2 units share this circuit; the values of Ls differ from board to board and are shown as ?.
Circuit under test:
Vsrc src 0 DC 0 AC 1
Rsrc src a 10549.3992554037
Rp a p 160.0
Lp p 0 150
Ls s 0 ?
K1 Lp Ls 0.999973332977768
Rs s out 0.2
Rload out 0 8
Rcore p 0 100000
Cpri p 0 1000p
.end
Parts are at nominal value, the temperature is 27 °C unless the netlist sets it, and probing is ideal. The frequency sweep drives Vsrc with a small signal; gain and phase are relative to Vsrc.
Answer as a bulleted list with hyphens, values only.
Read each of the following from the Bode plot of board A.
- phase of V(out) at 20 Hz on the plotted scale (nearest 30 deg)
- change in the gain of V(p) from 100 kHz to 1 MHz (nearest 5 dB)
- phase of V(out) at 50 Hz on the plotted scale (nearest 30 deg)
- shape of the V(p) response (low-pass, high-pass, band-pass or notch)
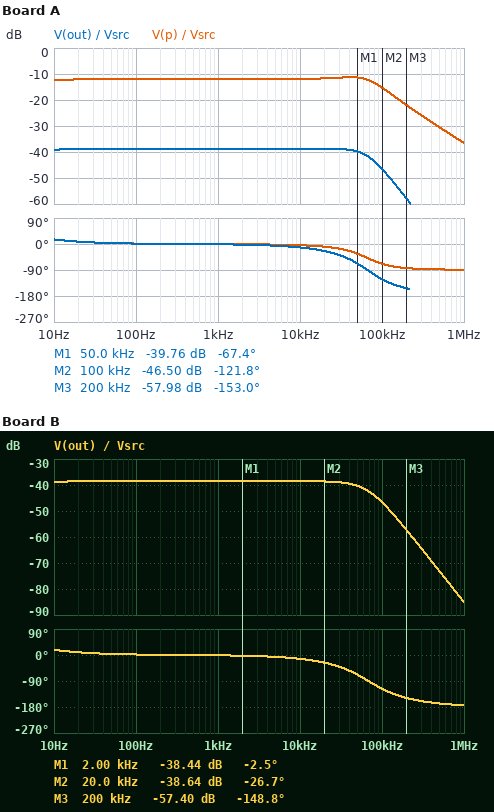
- 0 deg
- -20 dB
- 0 deg
- low-pass
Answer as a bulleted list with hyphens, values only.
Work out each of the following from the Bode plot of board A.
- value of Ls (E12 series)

- 330 mH
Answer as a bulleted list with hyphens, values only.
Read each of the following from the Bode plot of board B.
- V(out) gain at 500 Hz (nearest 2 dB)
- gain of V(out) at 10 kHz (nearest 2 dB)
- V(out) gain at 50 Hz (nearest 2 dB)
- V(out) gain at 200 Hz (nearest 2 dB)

- -38 dB
- -38 dB
- -38 dB
- -38 dB
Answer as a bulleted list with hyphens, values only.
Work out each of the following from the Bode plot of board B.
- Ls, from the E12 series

- 270 mH
